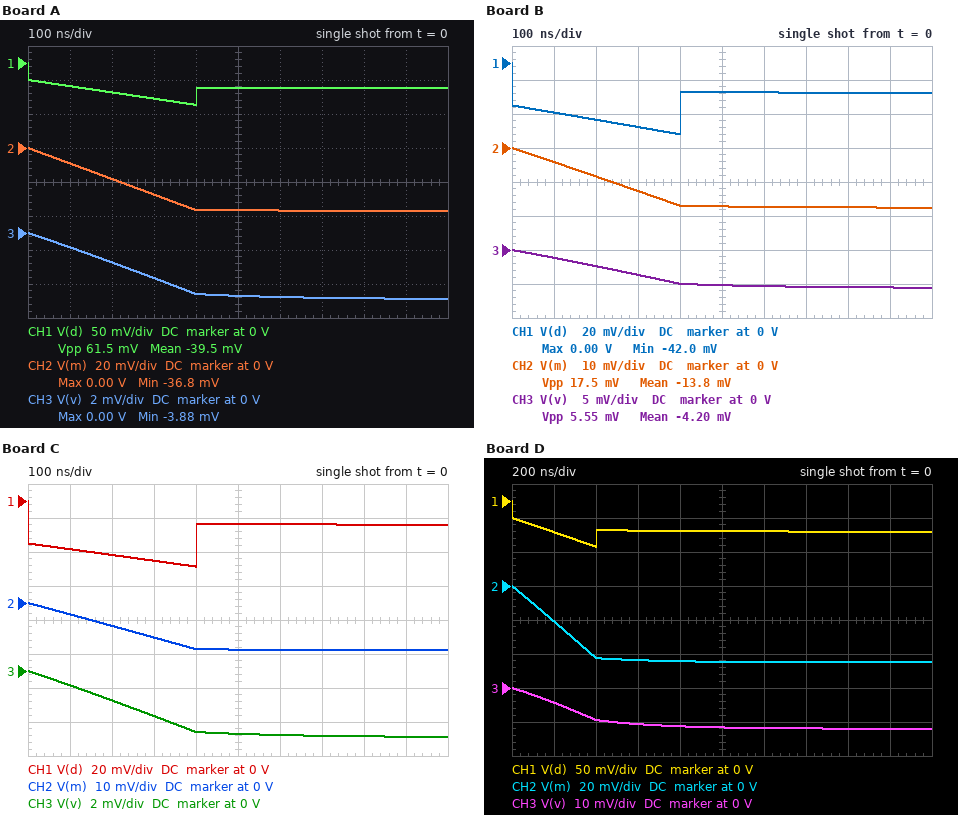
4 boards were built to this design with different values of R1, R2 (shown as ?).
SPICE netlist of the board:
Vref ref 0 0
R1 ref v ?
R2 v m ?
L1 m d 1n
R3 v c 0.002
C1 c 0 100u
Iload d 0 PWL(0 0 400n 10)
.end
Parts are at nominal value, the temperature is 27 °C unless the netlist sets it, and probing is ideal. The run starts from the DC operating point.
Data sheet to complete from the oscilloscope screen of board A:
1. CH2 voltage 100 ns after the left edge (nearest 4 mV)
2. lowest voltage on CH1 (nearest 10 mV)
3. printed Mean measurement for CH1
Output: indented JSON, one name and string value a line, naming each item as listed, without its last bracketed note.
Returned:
{
  "CH2 voltage 100 ns after the left edge": "-8 mV",
  "lowest voltage on CH1": "-60 mV",
  "printed Mean measurement for CH1": "-39.5 mV"
}
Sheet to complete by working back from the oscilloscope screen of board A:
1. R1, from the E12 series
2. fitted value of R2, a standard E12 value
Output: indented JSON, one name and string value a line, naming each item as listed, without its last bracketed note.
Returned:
{
  "R1, from the E12 series": "390 µΩ",
  "fitted value of R2, a standard E12 value": "3.3 mΩ"
}
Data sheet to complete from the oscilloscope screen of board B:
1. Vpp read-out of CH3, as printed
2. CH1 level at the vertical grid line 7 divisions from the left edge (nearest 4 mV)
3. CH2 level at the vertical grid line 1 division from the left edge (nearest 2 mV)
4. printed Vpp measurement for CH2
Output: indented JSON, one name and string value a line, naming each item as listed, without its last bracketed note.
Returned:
{
  "Vpp read-out of CH3, as printed": "5.55 mV",
  "CH1 level at the vertical grid line 7 divisions from the left edge": "-16 mV",
  "CH2 level at the vertical grid line 1 division from the left edge": "-4 mV",
  "printed Vpp measurement for CH2": "17.5 mV"
}
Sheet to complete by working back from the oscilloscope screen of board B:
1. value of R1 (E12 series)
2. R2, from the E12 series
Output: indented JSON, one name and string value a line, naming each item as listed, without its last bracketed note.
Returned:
{
  "value of R1": "560 µΩ",
  "R2, from the E12 series": "1.2 mΩ"
}
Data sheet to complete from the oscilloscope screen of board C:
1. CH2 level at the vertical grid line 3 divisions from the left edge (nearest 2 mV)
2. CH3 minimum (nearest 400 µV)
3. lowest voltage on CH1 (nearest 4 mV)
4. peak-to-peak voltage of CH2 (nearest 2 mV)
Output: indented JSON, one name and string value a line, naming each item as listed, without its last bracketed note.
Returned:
{
  "CH2 level at the vertical grid line 3 divisions from the left edge": "-10 mV",
  "CH3 minimum": "-4.0 mV",
  "lowest voltage on CH1": "-40 mV",
  "peak-to-peak voltage of CH2": "14 mV"
}
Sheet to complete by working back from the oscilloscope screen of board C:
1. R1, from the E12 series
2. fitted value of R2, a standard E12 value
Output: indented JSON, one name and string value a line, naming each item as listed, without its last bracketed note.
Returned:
{
  "R1, from the E12 series": "390 µΩ",
  "fitted value of R2, a standard E12 value": "1 mΩ"
}
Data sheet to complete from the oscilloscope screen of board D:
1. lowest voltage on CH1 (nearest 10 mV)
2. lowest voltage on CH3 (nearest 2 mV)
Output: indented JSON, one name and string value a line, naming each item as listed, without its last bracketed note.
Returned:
{
  "lowest voltage on CH1": "-70 mV",
  "lowest voltage on CH3": "-12 mV"
}
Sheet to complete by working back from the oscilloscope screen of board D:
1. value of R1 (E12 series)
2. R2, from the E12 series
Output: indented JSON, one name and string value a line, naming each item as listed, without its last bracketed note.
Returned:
{
  "value of R1": "1.2 mΩ",
  "R2, from the E12 series": "3.3 mΩ"
}
